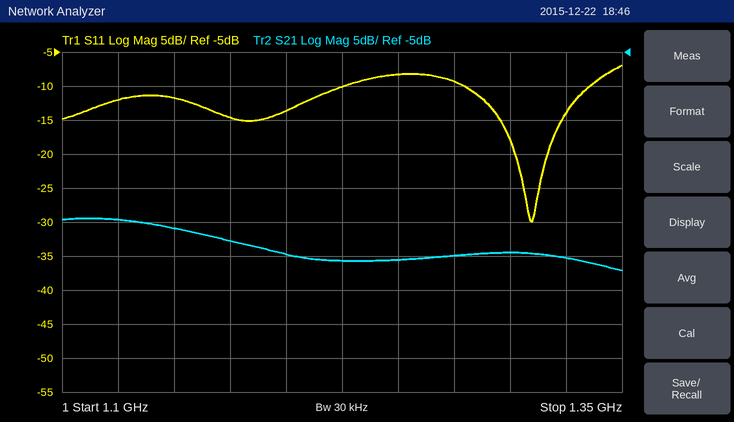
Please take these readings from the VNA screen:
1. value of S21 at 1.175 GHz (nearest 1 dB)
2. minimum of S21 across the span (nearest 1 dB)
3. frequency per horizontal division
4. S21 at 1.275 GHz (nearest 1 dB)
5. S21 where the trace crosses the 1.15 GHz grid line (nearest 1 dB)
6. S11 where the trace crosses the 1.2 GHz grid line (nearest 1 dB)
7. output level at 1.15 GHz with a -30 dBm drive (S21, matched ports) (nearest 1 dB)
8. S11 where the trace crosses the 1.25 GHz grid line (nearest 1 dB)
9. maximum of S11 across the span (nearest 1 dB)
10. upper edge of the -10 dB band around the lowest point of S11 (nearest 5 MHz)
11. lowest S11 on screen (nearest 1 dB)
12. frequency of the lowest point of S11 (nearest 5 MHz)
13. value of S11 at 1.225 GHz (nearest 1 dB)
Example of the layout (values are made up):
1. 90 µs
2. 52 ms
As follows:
1. -33 dB
2. -37 dB
3. 25 MHz
4. -35 dB
5. -31 dB
6. -14 dB
7. -61 dBm
8. -8 dB
9. -7 dB
10. 1.335 GHz
11. -30 dB
12. 1.310 GHz
13. -10 dB
